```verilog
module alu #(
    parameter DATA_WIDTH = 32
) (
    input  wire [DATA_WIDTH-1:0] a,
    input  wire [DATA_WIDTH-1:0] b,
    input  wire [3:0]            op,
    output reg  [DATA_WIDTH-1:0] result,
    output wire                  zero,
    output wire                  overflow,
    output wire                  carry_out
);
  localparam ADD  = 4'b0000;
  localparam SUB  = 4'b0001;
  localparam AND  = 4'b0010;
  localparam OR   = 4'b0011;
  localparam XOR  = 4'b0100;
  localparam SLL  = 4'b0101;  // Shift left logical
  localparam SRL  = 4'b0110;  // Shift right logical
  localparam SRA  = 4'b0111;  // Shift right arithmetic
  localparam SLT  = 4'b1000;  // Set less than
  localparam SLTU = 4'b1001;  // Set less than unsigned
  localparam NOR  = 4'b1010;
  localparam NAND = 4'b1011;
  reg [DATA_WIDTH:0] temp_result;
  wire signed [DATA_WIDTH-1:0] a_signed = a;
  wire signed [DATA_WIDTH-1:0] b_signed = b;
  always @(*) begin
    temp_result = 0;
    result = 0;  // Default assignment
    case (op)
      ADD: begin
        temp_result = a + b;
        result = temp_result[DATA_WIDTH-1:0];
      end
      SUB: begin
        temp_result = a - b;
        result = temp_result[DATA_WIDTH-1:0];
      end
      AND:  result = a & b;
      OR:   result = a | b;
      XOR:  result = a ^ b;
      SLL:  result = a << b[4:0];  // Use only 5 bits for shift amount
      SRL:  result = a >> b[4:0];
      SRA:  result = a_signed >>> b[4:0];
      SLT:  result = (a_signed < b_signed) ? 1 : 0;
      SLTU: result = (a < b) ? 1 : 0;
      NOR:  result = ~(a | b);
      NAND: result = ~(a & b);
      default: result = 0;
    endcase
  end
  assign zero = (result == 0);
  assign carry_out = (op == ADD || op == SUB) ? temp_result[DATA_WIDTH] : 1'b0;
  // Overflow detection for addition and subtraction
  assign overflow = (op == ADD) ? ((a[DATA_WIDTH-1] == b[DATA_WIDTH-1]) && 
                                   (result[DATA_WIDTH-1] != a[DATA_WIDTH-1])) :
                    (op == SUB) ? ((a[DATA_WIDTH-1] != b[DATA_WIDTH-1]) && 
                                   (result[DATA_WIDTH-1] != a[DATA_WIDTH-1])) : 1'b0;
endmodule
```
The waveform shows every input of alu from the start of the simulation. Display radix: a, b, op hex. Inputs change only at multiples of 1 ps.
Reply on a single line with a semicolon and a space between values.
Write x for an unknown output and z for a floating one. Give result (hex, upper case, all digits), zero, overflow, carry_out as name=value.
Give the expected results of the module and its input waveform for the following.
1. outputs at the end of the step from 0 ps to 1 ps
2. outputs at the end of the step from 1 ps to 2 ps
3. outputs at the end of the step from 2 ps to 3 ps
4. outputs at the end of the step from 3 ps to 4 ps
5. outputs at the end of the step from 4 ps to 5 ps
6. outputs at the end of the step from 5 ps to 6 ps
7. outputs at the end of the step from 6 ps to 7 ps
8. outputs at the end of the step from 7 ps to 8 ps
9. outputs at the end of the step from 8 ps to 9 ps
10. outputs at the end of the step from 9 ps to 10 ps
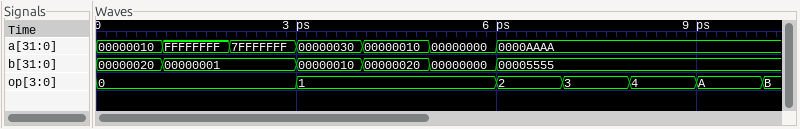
result=00000030, zero=0, overflow=0, carry_out=0; result=00000000, zero=1, overflow=0, carry_out=1; result=80000000, zero=0, overflow=1, carry_out=0; result=00000020, zero=0, overflow=0, carry_out=0; result=FFFFFFF0, zero=0, overflow=0, carry_out=1; result=00000000, zero=1, overflow=0, carry_out=0; result=00000000, zero=1, overflow=0, carry_out=0; result=0000FFFF, zero=0, overflow=0, carry_out=0; result=0000FFFF, zero=0, overflow=0, carry_out=0; result=FFFF0000, zero=0, overflow=0, carry_out=0
